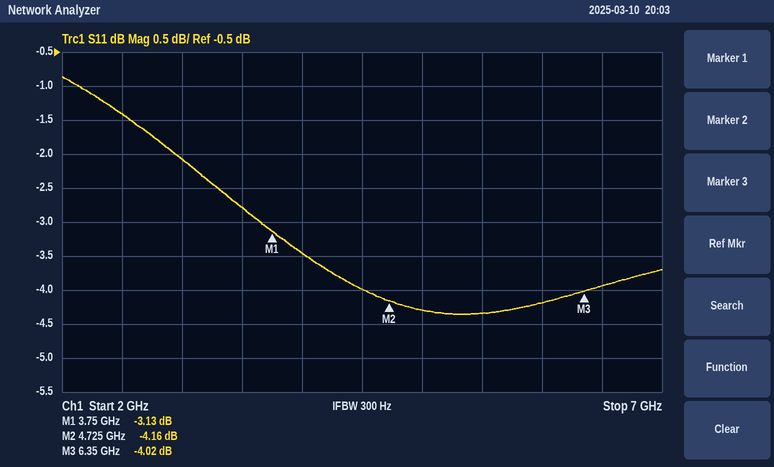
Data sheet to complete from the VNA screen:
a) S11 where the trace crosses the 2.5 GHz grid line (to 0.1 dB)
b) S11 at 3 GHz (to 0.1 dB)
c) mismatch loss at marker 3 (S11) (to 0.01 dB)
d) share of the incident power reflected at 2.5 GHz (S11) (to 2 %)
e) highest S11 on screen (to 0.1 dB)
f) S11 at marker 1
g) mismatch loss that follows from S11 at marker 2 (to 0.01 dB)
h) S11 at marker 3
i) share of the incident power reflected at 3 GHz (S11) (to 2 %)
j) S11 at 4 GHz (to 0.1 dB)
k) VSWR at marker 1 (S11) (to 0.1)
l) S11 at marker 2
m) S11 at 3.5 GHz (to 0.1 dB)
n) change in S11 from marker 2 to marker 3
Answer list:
-1.4 dB
-2.1 dB
2.19 dB
72 %
-0.9 dB
-3.13 dB
2.10 dB
-4.02 dB
62 %
-3.5 dB
5.6
-4.16 dB
-2.8 dB
0.14 dB
